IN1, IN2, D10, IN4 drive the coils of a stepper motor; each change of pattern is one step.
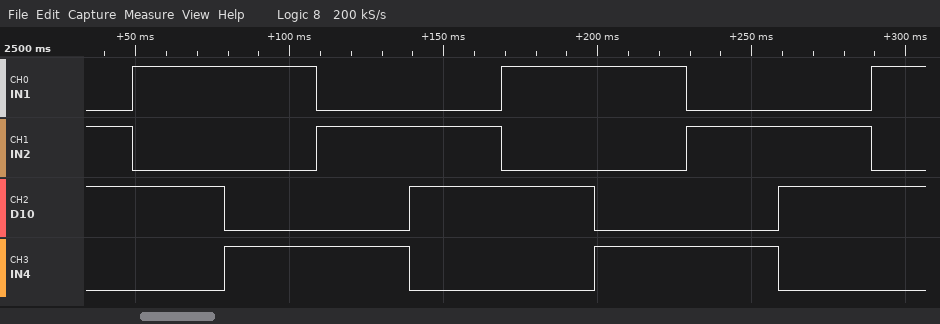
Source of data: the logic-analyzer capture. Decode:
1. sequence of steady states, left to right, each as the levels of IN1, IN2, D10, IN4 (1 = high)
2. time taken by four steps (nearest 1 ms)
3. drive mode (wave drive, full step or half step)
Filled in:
0110 1010 1001 0101 0110 1010 1001 0101 0110 1010
120 ms
full step
